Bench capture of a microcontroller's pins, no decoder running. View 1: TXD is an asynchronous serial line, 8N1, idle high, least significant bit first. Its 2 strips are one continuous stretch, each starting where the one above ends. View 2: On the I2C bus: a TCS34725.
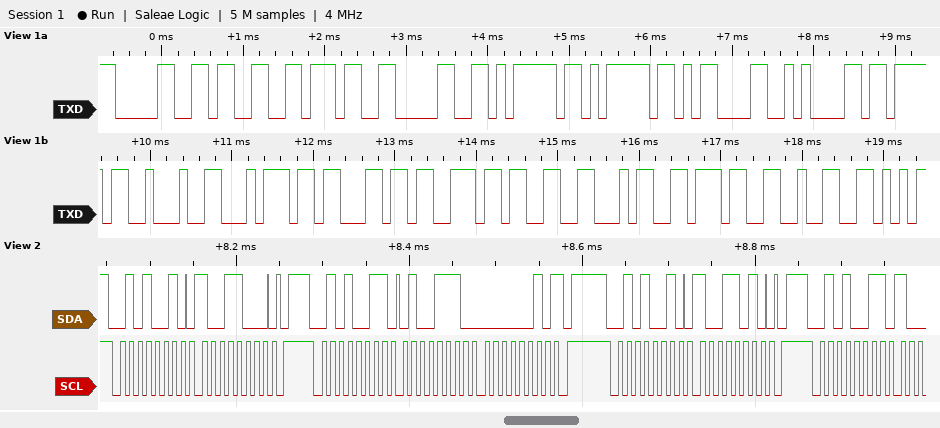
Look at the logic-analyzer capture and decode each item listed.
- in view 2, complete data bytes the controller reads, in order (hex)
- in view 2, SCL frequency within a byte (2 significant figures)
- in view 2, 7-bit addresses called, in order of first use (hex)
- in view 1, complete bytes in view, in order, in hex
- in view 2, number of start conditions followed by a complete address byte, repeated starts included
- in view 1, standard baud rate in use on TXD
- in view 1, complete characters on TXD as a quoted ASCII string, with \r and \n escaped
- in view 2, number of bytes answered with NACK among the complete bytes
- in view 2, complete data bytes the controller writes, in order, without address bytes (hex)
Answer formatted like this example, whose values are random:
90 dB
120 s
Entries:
4E 02
100 kHz
0x29
30 33 37 30 7D 7D 0D 0A 7B 22 74 63 73 33 34 37 32
4
9600 baud
"0370}}\r\n{\"tcs3472"
1
98 9A
